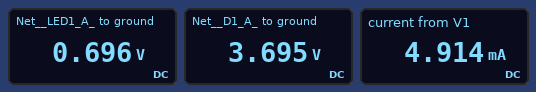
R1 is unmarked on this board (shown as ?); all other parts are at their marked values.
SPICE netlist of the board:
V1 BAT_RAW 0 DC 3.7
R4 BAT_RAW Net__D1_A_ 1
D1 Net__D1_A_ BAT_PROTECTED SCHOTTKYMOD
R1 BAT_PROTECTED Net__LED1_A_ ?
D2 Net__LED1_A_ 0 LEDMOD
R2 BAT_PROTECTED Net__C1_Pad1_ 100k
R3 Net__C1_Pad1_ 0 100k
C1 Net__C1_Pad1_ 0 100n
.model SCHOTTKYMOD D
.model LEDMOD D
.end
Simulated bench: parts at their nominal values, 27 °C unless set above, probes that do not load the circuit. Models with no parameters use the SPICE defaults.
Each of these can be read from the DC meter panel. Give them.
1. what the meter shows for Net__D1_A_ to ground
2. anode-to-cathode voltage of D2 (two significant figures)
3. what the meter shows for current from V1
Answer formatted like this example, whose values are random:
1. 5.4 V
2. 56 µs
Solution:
1. 3.695 V
2. 700 mV
3. 4.914 mA
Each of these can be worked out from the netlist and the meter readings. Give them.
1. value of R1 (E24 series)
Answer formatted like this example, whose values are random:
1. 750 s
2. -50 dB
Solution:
1. 470 Ω
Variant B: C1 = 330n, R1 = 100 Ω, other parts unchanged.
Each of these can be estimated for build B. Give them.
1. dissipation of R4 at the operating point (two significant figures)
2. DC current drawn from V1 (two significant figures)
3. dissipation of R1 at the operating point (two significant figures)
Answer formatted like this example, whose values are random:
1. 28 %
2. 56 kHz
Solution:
1. 490 µW
2. 22 mA
3. 49 mW
